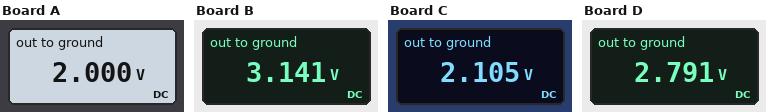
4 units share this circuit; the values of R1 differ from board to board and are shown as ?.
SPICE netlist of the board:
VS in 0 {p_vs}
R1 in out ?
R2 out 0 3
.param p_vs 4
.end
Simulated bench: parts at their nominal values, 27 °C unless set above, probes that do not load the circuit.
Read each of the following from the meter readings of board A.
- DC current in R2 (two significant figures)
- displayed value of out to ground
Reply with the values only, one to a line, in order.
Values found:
670 mA
2.000 V
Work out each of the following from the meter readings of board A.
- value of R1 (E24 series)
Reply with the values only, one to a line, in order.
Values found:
3 Ω
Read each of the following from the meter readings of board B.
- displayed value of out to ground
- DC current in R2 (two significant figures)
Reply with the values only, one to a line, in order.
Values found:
3.141 V
1.0 A
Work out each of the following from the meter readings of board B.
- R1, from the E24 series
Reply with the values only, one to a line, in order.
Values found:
0.82 Ω
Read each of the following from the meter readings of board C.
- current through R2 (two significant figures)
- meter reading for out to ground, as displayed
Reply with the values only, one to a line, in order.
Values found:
700 mA
2.105 V
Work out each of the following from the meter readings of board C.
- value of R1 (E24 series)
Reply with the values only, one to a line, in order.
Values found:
2.7 Ω
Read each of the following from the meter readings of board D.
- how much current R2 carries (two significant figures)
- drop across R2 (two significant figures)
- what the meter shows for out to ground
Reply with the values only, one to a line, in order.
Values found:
930 mA
2.8 V
2.791 V
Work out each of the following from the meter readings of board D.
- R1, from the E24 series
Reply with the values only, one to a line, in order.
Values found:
1.3 Ω
